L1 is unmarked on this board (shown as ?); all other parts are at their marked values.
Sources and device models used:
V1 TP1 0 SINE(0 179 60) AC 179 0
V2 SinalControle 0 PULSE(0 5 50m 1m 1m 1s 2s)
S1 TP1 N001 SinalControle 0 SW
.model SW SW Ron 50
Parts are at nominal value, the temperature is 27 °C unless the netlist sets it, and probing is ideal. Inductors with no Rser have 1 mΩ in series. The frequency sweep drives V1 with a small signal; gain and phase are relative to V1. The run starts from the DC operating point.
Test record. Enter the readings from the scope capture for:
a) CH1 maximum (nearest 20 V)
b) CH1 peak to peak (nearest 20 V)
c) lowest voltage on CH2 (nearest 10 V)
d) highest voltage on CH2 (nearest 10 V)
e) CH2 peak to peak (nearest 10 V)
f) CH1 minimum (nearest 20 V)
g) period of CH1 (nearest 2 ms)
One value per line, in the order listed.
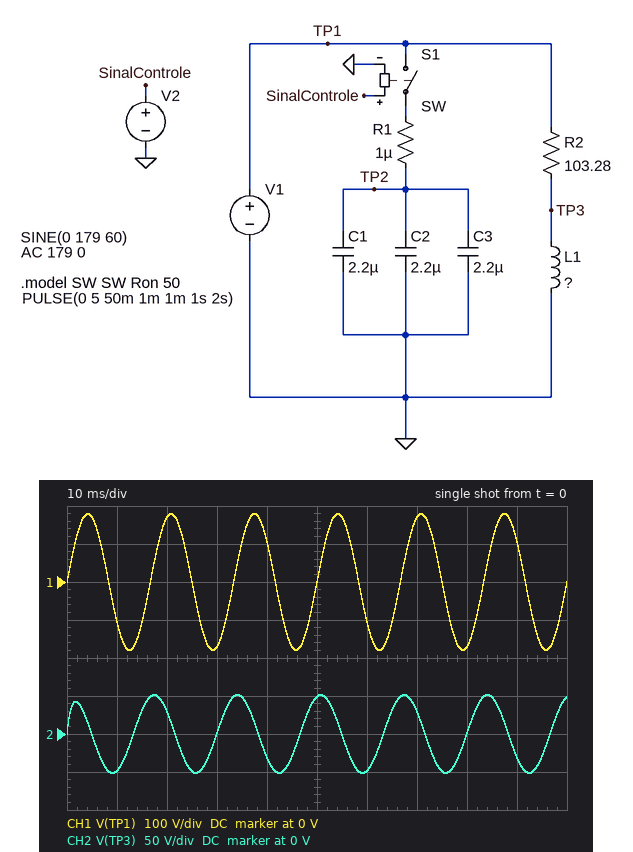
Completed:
180 V
360 V
-50 V
50 V
100 V
-180 V
16 ms
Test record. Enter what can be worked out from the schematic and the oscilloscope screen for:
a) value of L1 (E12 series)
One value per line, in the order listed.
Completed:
82 mH
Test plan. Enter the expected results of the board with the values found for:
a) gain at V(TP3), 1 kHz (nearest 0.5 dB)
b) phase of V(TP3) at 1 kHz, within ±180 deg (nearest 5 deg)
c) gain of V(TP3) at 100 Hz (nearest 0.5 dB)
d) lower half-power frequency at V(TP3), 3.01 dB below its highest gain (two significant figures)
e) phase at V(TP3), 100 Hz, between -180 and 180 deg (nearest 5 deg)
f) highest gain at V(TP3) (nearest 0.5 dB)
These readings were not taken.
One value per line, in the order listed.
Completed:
0 dB
10 deg
-7.0 dB
200 Hz
65 deg
0 dB
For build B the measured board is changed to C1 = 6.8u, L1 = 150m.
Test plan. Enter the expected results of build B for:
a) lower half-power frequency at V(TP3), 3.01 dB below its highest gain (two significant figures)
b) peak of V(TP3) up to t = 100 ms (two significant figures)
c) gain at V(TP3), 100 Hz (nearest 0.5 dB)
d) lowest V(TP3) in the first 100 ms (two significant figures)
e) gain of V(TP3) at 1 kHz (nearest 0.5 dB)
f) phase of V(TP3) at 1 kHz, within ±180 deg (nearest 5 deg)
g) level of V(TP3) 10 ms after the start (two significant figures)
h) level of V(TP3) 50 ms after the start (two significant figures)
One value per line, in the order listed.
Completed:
110 Hz
86 V
-3.5 dB
-86 V
0 dB
5 deg
-85 V
75 V
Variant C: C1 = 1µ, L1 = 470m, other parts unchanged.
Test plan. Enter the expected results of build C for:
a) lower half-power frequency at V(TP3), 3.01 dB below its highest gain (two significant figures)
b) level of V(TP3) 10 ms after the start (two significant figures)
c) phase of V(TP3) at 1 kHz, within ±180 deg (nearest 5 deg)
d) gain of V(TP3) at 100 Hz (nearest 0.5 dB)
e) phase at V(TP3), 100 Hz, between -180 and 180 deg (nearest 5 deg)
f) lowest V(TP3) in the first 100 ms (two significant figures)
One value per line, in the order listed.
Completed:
35 Hz
-150 V
0 deg
-0.5 dB
20 deg
-160 V
